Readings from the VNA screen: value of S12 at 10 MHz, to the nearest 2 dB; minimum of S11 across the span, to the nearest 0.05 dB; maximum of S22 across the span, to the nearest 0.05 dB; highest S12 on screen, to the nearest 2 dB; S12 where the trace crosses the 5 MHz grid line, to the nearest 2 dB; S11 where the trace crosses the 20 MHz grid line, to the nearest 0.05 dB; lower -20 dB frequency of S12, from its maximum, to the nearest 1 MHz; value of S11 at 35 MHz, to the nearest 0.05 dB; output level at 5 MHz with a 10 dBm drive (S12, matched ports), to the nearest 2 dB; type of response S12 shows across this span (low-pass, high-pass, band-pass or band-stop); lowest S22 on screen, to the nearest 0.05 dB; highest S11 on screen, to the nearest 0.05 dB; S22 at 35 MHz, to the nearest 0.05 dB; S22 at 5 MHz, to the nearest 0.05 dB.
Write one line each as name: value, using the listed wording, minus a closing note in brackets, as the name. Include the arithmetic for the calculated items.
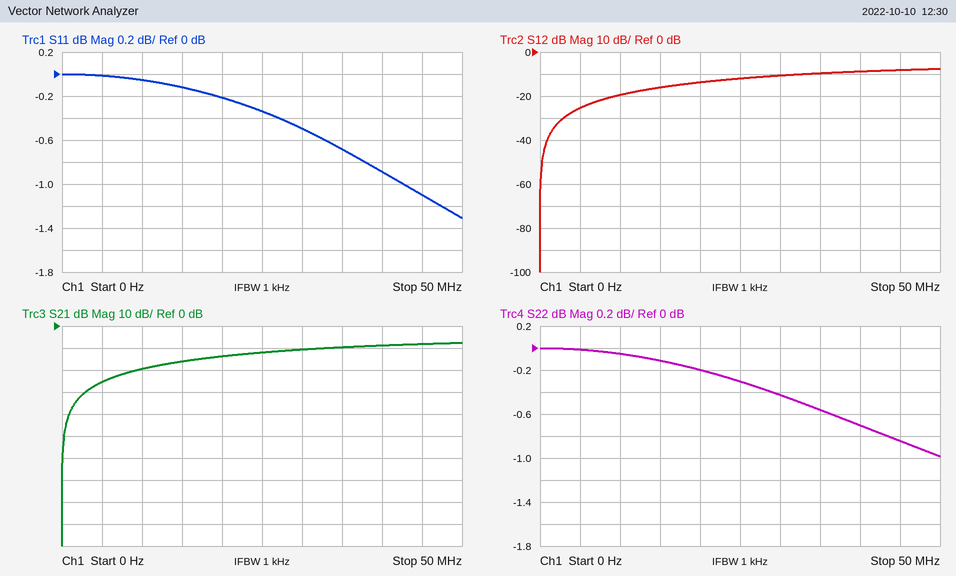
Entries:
value of S12 at 10 MHz, to the nearest 2 dB: -20 dB
minimum of S11 across the span, to the nearest 0.05 dB: -1.30 dB
maximum of S22 across the span, to the nearest 0.05 dB: 0.00 dB
highest S12 on screen, to the nearest 2 dB: -8 dB
S12 where the trace crosses the 5 MHz grid line, to the nearest 2 dB: -26 dB
S11 where the trace crosses the 20 MHz grid line, to the nearest 0.05 dB: -0.20 dB
lower -20 dB frequency of S12, from its maximum, to the nearest 1 MHz: 4 MHz
value of S11 at 35 MHz, to the nearest 0.05 dB: -0.70 dB
output level at 5 MHz with a 10 dBm drive (S12, matched ports), to the nearest 2 dB: 10 dBm + (-26 dB) = -16 dBm
type of response S12 shows across this span: high-pass
lowest S22 on screen, to the nearest 0.05 dB: -1.00 dB
highest S11 on screen, to the nearest 0.05 dB: 0.00 dB
S22 at 35 MHz, to the nearest 0.05 dB: -0.55 dB
S22 at 5 MHz, to the nearest 0.05 dB: 0.00 dB
